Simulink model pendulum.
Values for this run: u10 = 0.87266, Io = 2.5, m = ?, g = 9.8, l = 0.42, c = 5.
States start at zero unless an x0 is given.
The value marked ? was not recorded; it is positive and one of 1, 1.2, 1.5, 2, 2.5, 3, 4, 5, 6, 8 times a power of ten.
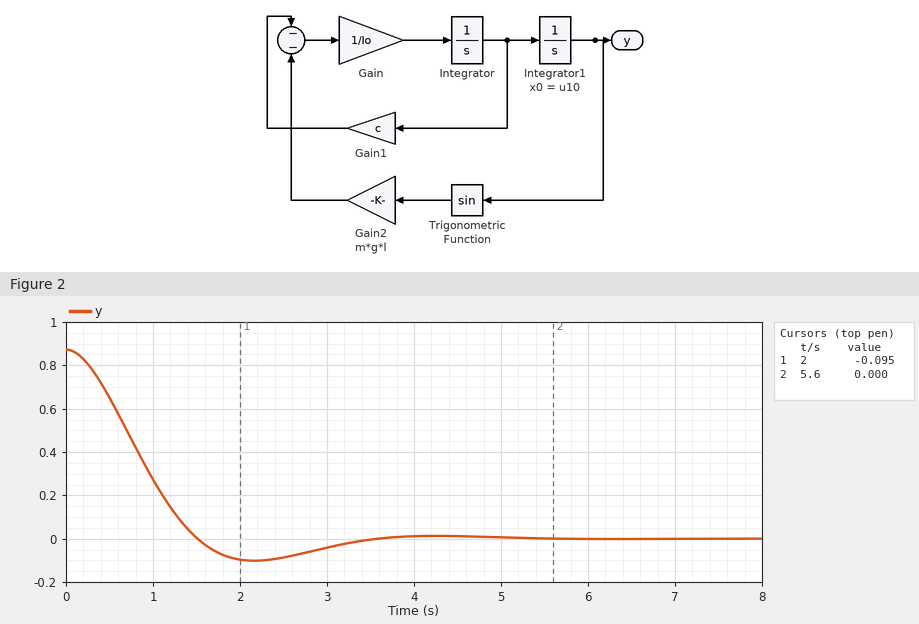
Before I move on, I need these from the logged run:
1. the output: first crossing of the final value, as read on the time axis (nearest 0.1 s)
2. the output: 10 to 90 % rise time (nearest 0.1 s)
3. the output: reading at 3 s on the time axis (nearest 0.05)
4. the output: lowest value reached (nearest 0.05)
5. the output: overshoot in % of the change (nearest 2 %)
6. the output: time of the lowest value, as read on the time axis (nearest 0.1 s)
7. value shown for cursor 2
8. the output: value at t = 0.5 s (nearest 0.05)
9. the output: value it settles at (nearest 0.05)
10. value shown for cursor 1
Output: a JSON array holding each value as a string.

["1.5 s", "1.0 s", "-0.05", "-0.10", "12 %", "2.2 s", "0.000", "0.65", "0.00", "-0.095"]
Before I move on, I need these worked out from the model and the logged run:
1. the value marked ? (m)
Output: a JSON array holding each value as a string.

["2"]
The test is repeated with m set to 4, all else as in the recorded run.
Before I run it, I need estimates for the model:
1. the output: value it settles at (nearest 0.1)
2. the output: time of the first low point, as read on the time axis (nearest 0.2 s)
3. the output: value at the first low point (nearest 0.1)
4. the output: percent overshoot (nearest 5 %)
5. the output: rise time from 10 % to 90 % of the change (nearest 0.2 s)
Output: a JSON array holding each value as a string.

["0.0", "1.4 s", "-0.2", "25 %", "0.6 s"]
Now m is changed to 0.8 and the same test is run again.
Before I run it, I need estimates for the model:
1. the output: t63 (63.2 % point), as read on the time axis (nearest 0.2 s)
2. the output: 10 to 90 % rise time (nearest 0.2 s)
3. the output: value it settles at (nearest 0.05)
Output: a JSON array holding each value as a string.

["1.8 s", "2.6 s", "0.00"]
